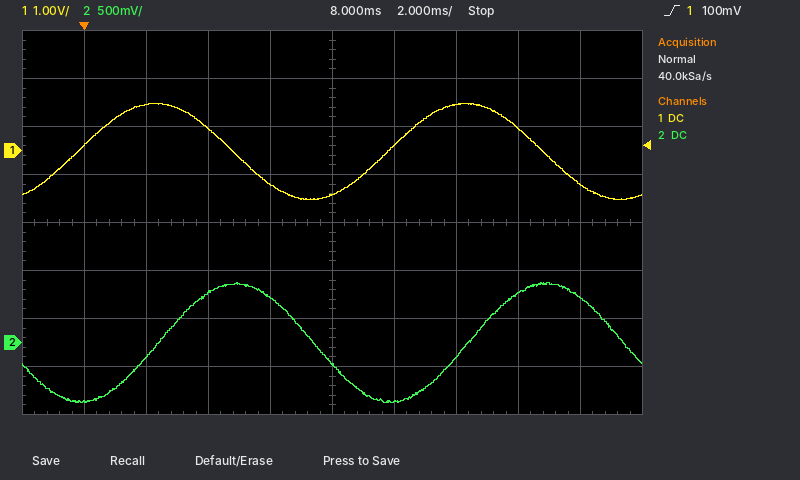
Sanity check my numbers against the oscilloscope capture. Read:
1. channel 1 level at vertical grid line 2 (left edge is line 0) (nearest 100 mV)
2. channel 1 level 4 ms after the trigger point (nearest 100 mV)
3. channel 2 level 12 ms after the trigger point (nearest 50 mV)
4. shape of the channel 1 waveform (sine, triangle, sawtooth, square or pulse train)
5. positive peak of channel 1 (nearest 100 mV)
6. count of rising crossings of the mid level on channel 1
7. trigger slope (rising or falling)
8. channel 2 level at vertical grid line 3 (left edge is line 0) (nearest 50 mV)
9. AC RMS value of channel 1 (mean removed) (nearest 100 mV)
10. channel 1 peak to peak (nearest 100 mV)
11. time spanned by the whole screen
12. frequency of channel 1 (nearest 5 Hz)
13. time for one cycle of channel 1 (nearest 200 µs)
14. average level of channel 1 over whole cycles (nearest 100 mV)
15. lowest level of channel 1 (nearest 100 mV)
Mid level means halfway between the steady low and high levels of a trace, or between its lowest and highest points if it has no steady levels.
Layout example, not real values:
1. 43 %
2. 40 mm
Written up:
1. 1.0 V
2. 500 mV
3. -150 mV
4. sine
5. 1.0 V
6. 2
7. rising
8. 500 mV
9. 700 mV
10. 2.0 V
11. 20 ms
12. 100 Hz
13. 10.0 ms
14. 0.0 V
15. -1.0 V
